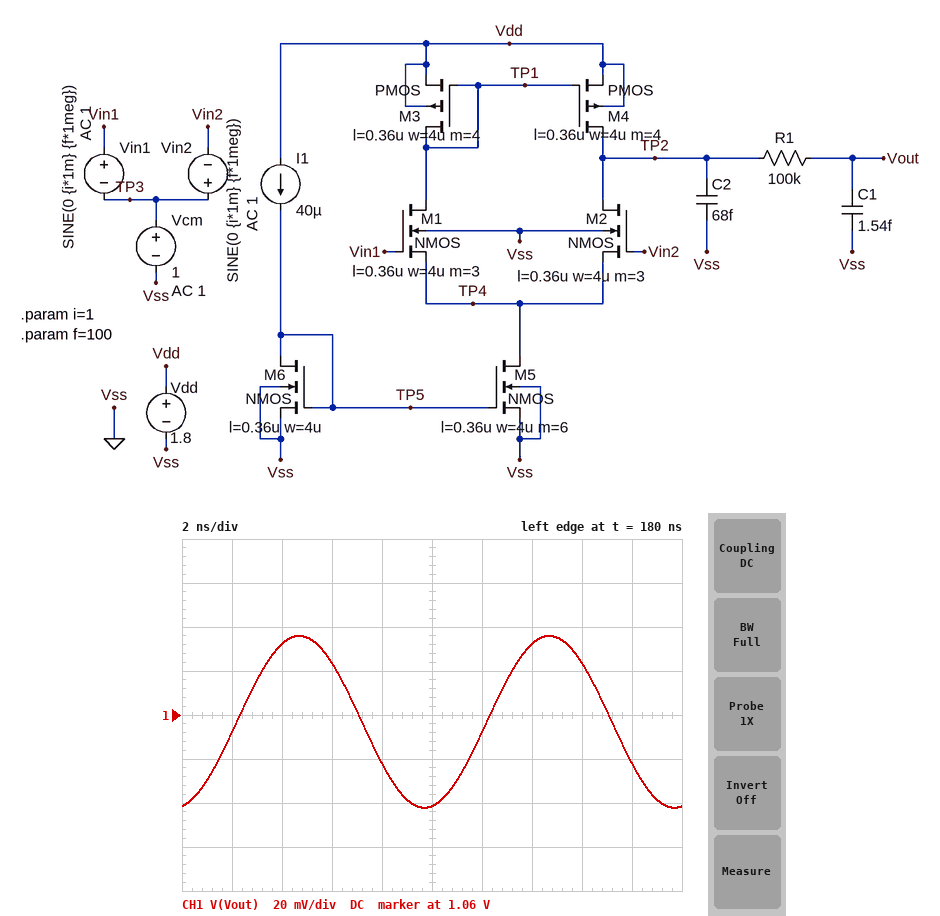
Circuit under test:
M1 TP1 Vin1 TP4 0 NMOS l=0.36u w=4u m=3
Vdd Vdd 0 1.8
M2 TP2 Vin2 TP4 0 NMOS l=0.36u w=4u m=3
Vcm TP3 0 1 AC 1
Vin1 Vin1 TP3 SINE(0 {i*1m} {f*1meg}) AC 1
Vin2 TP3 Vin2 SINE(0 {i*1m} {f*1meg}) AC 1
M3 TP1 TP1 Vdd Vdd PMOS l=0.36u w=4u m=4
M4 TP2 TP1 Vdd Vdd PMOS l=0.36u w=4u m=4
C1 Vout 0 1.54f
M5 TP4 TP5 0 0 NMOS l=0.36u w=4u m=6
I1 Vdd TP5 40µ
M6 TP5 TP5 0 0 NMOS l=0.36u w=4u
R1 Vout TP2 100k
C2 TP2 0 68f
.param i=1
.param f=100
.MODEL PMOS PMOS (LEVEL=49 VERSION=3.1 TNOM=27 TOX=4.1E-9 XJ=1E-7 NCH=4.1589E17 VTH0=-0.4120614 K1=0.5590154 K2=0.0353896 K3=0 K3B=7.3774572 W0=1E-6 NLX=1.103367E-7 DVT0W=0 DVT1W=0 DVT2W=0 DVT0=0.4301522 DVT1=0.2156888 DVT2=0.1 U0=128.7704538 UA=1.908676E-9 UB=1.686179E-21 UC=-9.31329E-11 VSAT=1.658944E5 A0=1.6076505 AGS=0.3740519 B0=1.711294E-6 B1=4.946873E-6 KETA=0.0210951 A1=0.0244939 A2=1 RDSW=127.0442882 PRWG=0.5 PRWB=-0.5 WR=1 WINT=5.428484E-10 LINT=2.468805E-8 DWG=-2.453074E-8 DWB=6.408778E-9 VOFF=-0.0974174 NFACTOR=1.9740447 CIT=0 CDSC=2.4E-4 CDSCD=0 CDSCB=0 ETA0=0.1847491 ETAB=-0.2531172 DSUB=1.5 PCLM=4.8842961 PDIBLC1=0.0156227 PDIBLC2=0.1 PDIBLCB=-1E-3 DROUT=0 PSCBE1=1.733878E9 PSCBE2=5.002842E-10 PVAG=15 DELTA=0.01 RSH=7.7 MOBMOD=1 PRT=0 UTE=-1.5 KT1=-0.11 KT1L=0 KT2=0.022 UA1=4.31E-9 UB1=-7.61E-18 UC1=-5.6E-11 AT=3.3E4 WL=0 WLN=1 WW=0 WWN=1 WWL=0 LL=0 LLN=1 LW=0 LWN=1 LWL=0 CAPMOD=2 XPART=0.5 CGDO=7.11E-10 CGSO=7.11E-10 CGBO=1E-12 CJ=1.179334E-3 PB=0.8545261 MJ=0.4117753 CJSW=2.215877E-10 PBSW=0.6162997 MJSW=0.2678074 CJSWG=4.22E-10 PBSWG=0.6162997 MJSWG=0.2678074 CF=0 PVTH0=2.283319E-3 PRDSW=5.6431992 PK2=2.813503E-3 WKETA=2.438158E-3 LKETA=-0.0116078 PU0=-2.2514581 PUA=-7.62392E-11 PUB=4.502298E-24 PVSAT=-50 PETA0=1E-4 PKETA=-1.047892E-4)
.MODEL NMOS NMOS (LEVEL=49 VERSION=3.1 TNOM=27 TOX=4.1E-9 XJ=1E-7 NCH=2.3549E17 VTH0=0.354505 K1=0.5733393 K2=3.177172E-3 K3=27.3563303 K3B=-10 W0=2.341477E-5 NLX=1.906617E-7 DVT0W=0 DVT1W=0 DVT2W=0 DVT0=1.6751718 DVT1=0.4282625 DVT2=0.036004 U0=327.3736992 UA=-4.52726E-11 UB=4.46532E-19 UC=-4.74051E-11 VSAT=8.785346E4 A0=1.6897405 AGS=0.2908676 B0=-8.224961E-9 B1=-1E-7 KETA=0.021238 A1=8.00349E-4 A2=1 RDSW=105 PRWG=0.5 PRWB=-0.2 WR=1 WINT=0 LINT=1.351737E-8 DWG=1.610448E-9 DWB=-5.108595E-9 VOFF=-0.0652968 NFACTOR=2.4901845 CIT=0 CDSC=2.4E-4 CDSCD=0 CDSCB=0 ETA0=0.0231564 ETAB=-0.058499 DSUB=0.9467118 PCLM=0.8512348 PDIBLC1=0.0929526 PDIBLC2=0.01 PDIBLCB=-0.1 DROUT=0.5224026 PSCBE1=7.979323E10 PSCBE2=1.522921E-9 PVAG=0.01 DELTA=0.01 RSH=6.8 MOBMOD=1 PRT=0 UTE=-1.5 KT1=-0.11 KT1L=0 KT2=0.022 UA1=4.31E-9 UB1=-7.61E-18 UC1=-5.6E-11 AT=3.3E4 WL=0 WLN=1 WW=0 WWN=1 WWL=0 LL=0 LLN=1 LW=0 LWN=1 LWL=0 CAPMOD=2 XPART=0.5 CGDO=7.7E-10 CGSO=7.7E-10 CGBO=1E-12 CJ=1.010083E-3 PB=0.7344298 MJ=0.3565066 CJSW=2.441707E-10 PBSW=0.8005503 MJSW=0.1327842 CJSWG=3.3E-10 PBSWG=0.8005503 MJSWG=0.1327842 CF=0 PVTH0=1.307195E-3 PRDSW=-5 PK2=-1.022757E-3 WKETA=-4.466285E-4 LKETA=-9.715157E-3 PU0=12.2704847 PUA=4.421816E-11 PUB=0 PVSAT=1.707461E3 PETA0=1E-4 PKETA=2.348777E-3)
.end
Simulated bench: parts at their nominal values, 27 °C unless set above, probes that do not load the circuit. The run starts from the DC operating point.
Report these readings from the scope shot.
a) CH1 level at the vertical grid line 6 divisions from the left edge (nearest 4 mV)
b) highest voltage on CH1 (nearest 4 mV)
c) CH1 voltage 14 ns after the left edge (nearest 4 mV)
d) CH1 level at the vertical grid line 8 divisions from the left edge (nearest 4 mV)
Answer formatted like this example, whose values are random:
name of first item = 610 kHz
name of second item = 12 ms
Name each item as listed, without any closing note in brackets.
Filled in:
CH1 level at the vertical grid line 6 divisions from the left edge = 1.052 V
highest voltage on CH1 = 1.096 V
CH1 voltage 14 ns after the left edge = 1.092 V
CH1 level at the vertical grid line 8 divisions from the left edge = 1.084 V
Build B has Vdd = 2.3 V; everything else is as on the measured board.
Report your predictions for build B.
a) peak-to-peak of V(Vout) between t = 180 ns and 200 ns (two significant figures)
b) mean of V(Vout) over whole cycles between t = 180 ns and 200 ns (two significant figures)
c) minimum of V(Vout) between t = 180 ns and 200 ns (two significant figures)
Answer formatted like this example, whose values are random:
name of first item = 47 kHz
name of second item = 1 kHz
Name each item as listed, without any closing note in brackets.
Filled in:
peak-to-peak of V(Vout) between t = 180 ns and 200 ns = 79 mV
mean of V(Vout) over whole cycles between t = 180 ns and 200 ns = 1.6 V
minimum of V(Vout) between t = 180 ns and 200 ns = 1.5 V
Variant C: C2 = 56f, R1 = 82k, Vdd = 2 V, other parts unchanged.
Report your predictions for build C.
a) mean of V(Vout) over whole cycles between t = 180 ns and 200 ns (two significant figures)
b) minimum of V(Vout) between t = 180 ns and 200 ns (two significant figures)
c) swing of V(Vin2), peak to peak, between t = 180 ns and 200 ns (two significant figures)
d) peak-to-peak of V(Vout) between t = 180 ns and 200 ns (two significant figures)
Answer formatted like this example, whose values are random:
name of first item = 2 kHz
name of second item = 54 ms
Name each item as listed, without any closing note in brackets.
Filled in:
mean of V(Vout) over whole cycles between t = 180 ns and 200 ns = 1.3 V
minimum of V(Vout) between t = 180 ns and 200 ns = 1.2 V
swing of V(Vin2), peak to peak, between t = 180 ns and 200 ns = 2.0 mV
peak-to-peak of V(Vout) between t = 180 ns and 200 ns = 88 mV
